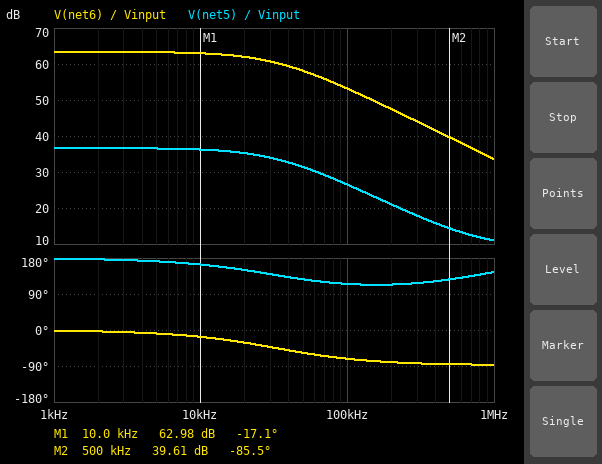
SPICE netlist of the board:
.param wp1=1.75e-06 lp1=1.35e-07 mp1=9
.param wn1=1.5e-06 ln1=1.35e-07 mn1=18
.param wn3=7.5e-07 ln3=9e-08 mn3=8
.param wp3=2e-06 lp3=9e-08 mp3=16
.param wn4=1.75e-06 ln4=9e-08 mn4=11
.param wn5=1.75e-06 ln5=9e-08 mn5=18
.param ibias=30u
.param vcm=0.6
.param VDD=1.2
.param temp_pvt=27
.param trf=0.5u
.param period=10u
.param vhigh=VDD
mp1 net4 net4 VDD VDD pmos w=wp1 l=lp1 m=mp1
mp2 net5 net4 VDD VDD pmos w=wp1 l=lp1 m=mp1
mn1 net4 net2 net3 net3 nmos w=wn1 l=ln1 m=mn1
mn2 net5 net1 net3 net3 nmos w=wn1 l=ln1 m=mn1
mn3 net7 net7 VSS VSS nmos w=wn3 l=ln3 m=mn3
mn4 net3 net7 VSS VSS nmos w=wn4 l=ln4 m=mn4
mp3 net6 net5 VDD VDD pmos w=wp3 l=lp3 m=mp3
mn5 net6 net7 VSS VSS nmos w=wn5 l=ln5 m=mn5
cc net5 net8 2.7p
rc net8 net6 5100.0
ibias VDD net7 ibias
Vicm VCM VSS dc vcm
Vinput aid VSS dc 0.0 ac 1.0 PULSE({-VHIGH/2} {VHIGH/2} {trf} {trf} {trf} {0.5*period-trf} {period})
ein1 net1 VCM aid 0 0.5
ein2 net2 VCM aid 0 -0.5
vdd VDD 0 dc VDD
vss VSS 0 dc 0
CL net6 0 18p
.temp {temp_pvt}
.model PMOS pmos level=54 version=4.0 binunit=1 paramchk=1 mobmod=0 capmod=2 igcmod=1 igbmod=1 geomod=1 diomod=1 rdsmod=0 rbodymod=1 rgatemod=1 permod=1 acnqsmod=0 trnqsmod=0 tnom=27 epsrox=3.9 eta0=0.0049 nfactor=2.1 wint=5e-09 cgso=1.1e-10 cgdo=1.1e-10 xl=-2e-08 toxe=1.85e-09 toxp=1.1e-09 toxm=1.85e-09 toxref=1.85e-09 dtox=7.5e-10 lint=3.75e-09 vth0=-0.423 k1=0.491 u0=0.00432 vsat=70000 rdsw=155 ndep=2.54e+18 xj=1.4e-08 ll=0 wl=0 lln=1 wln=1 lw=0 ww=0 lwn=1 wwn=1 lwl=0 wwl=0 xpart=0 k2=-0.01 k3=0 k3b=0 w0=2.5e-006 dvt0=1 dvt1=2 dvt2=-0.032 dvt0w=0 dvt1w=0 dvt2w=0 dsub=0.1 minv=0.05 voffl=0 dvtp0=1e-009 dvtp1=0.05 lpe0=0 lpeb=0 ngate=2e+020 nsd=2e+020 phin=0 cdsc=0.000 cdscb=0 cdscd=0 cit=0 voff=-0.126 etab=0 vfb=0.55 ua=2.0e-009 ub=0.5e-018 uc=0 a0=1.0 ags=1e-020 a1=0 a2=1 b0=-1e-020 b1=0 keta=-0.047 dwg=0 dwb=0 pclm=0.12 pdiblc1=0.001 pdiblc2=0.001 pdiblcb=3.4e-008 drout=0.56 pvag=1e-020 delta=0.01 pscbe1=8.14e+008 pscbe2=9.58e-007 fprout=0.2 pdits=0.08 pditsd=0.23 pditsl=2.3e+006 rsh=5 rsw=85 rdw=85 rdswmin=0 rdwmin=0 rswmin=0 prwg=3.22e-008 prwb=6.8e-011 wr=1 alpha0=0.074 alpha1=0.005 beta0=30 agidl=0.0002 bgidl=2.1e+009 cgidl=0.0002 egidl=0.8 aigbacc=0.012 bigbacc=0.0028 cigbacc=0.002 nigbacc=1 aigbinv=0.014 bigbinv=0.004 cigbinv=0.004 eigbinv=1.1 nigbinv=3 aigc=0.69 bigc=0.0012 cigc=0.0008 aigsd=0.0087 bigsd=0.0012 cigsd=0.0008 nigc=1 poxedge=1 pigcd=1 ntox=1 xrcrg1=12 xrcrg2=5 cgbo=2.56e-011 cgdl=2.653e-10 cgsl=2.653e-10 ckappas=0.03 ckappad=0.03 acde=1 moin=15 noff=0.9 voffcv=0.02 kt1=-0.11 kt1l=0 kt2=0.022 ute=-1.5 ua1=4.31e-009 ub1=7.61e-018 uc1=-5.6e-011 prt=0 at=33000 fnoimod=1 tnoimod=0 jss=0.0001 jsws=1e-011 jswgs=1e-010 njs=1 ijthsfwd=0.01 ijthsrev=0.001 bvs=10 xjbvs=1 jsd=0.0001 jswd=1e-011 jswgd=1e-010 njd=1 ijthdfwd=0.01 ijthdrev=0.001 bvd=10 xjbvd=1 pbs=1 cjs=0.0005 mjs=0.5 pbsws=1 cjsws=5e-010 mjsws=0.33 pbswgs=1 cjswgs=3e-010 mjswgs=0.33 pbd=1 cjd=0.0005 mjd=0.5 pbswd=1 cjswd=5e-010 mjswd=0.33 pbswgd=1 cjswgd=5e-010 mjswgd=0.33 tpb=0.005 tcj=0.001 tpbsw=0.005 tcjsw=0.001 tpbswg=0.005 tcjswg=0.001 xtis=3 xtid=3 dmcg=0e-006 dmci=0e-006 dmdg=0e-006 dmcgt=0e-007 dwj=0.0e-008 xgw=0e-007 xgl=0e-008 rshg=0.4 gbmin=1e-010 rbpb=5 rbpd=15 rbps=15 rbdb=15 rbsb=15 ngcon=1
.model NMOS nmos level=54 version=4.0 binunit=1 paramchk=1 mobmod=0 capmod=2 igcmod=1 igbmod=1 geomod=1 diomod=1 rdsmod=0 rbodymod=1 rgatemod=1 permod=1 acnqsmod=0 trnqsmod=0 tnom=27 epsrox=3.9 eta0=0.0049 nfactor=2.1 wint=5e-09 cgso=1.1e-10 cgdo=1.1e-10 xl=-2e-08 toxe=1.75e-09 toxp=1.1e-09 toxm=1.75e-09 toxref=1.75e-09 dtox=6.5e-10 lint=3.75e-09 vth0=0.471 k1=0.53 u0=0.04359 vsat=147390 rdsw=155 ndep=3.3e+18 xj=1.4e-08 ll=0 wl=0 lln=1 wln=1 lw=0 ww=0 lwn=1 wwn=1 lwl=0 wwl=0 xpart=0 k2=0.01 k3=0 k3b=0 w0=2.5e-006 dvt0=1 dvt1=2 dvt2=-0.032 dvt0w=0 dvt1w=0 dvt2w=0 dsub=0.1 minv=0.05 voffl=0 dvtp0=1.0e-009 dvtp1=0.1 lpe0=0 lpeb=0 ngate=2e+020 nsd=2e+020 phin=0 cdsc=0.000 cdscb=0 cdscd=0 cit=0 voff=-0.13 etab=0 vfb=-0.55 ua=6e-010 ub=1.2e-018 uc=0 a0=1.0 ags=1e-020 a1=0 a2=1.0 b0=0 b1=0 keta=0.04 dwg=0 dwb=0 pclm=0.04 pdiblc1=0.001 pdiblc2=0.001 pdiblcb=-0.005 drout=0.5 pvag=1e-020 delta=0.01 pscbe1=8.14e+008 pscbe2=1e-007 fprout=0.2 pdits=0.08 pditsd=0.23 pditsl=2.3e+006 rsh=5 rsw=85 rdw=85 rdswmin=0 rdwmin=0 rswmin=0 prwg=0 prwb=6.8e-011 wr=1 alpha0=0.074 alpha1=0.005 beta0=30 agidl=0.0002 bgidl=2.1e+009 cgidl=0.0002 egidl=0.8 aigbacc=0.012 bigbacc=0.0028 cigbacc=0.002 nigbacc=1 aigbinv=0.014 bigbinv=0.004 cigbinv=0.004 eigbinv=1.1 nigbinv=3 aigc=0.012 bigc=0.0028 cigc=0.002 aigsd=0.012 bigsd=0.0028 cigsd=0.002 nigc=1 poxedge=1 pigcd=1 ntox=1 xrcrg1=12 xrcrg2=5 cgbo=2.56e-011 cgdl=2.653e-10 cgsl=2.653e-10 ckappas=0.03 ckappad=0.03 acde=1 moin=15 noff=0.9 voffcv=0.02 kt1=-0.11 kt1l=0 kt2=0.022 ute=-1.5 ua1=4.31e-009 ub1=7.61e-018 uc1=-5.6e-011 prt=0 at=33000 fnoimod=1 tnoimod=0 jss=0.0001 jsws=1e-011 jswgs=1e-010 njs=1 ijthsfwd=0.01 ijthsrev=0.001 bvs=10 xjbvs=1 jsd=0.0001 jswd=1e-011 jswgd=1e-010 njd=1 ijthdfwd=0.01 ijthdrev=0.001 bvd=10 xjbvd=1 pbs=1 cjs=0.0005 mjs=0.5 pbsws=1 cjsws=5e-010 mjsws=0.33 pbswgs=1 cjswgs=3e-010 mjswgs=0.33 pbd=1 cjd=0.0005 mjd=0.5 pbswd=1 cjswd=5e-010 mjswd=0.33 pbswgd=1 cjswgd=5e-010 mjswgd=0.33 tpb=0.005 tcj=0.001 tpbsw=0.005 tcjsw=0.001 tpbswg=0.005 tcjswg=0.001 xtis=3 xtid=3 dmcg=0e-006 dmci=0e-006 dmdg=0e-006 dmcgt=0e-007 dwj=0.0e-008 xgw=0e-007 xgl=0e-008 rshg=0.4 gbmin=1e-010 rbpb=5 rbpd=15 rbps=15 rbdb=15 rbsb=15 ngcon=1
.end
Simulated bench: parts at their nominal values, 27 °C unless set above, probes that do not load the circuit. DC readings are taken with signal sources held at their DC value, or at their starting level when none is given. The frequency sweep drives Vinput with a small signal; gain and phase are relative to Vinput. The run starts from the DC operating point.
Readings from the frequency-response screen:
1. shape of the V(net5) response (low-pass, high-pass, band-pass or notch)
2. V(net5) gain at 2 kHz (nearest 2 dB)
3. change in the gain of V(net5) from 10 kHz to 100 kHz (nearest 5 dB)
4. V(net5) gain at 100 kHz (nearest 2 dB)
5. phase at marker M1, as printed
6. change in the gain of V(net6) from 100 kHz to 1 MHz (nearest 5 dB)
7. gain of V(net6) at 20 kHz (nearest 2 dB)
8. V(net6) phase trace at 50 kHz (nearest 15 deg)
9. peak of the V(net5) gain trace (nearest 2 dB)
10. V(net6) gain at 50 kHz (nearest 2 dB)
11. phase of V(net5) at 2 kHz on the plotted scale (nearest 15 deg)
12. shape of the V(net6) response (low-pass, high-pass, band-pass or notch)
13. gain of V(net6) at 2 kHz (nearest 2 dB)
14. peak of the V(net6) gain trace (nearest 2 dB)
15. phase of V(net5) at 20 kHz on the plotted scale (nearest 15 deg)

low-pass
36 dB
-10 dB
26 dB
-17.1 deg
-20 dB
62 dB
-60 deg
36 dB
58 dB
180 deg
low-pass
64 dB
64 dB
150 deg
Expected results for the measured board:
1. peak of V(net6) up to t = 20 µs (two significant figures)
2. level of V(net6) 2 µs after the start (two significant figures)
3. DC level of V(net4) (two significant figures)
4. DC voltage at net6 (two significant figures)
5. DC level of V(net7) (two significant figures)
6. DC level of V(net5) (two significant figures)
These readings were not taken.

1.2 V
1.2 V
680 mV
680 mV
410 mV
680 mV
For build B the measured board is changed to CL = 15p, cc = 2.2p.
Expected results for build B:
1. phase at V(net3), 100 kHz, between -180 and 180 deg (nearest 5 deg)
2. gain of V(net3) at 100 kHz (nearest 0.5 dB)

120 deg
-20.0 dB
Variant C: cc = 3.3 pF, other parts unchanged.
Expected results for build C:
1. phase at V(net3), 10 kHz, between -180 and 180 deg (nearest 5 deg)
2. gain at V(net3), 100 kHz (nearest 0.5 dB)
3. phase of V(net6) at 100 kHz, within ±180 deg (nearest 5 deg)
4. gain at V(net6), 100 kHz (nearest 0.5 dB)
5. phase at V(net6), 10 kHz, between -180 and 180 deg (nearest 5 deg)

160 deg
-23.0 dB
-75 deg
51.5 dB
-20 deg
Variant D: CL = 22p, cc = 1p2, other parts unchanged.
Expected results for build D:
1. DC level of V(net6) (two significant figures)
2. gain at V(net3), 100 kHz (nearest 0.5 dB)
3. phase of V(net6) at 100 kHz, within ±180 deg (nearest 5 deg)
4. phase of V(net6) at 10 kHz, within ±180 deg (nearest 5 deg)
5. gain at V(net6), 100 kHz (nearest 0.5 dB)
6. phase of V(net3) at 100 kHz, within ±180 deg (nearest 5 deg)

680 mV
-16.0 dB
-55 deg
-10 deg
58.5 dB
135 deg
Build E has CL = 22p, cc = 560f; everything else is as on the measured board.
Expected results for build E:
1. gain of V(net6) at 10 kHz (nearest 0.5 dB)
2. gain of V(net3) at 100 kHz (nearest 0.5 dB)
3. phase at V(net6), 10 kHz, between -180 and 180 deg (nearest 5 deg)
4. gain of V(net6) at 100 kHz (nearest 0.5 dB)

63.5 dB
-13.0 dB
-5 deg
61.5 dB
